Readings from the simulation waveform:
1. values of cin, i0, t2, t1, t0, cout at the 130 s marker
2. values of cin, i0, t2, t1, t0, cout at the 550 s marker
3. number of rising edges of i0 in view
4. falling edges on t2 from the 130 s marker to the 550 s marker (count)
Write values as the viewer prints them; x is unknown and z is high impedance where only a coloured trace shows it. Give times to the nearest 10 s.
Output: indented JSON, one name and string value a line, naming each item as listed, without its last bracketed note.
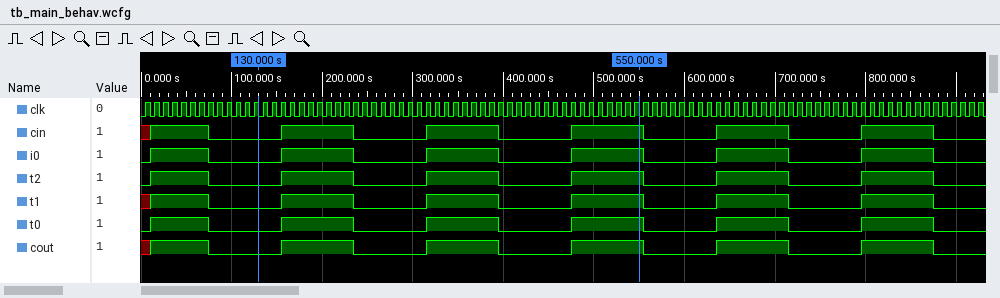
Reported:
{
  "values of cin, i0, t2, t1, t0, cout at the 130 s marker": "cin=0, i0=0, t2=0, t1=0, t0=0, cout=0",
  "values of cin, i0, t2, t1, t0, cout at the 550 s marker": "cin=1, i0=1, t2=1, t1=1, t0=1, cout=1",
  "number of rising edges of i0 in view": "6",
  "falling edges on t2 from the 130 s marker to the 550 s marker": "2"
}
